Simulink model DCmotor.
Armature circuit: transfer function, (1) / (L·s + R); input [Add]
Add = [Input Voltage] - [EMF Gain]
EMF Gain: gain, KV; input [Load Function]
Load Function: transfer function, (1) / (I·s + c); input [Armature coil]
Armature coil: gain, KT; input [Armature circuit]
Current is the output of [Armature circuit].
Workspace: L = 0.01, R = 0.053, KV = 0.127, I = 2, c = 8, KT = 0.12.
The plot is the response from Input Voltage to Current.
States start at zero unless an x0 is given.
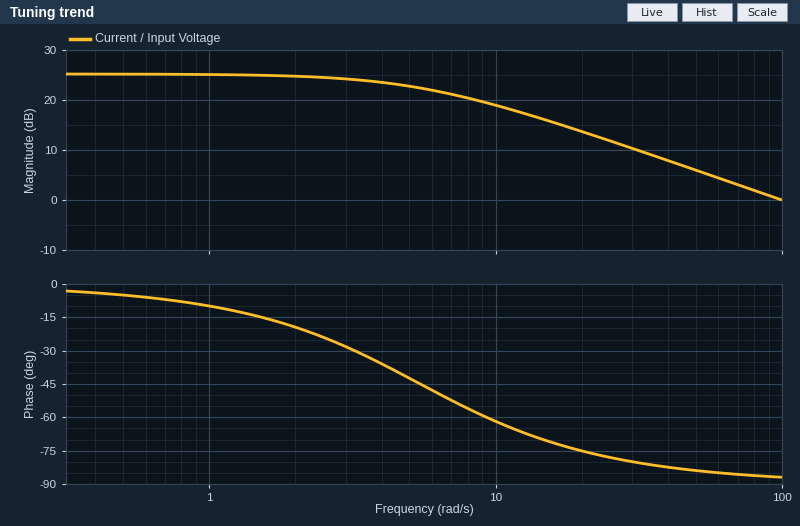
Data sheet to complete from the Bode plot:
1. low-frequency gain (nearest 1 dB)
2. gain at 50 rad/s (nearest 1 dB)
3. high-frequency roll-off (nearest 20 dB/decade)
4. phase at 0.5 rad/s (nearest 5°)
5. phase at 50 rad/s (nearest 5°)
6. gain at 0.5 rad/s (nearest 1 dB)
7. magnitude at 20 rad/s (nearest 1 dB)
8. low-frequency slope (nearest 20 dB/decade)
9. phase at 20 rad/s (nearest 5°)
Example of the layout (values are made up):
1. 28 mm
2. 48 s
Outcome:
1. 25 dB
2. 6 dB
3. -20 dB/decade
4. -5°
5. -85°
6. 25 dB
7. 14 dB
8. 0 dB/decade
9. -75°
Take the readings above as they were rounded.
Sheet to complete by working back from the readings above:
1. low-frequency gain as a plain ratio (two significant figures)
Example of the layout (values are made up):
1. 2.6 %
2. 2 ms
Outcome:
1. 18
